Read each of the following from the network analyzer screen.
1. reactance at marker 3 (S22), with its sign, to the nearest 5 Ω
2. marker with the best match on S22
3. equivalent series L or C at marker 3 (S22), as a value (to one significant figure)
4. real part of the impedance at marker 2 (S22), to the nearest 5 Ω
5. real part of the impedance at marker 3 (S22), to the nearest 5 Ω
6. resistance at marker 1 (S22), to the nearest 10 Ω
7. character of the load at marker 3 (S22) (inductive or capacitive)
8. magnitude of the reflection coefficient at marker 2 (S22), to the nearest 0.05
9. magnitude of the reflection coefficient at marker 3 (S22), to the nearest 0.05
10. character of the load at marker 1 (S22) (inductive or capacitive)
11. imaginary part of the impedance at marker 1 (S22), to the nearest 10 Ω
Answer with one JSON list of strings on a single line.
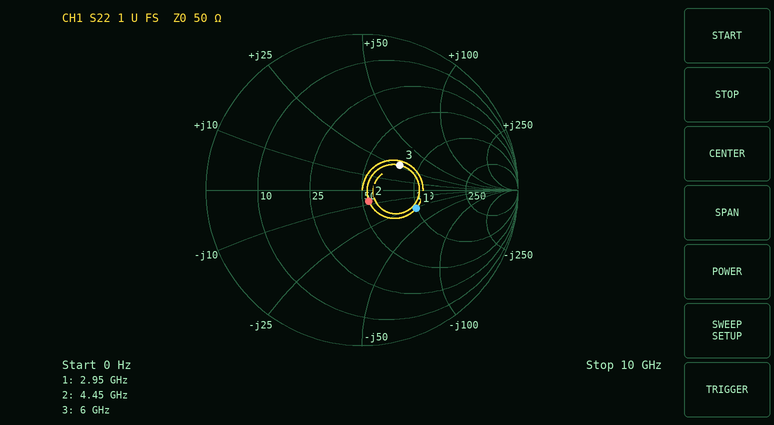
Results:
["+25 Ω", "marker 2", "700 pH", "55 Ω", "75 Ω", "100 Ω", "inductive", "0.10", "0.30", "capacitive", "-30 Ω"]
